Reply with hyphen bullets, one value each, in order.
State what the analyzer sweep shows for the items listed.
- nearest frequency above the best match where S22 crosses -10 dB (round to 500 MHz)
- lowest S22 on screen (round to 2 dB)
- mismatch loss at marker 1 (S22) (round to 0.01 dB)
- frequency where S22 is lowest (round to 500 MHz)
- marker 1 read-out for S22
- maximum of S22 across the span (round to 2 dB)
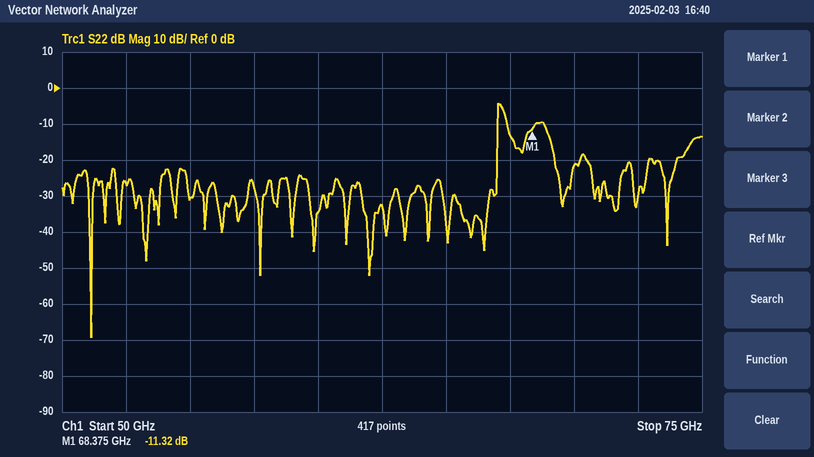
- 67.0 GHz
- -70 dB
- 0.33 dB
- 51.0 GHz
- -11.32 dB
- -4 dB
